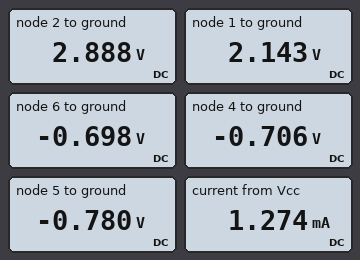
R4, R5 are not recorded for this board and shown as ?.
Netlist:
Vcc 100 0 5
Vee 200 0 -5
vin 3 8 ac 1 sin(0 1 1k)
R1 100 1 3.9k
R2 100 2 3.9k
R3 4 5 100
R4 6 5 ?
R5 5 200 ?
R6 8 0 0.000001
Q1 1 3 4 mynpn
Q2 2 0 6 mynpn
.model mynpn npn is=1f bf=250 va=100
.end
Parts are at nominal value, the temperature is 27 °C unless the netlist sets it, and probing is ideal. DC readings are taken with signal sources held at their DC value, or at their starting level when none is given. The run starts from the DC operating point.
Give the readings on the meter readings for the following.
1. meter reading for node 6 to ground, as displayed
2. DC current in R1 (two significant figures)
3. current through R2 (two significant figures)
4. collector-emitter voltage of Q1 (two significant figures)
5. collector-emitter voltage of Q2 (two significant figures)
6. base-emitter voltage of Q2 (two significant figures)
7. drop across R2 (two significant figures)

-0.698 V
730 µA
540 µA
2.8 V
3.6 V
700 mV
2.1 V
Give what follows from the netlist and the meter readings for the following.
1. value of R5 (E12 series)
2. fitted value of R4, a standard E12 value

3.3 kΩ
150 Ω
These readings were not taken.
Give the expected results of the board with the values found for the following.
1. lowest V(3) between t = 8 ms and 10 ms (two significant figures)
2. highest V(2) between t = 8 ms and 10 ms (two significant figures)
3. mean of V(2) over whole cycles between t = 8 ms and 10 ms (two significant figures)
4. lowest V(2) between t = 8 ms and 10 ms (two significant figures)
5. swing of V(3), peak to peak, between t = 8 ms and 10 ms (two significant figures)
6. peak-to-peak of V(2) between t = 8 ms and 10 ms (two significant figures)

-1.0 V
5.0 V
2.6 V
180 mV
2.0 V
4.8 V
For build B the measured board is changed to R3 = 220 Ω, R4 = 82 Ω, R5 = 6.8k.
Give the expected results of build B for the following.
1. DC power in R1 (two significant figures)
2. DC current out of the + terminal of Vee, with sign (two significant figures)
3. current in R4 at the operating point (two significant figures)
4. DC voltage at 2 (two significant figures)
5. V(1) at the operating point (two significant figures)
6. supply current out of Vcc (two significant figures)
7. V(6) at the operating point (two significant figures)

190 µW
-630 µA
410 µA
3.4 V
4.1 V
630 µA
-690 mV
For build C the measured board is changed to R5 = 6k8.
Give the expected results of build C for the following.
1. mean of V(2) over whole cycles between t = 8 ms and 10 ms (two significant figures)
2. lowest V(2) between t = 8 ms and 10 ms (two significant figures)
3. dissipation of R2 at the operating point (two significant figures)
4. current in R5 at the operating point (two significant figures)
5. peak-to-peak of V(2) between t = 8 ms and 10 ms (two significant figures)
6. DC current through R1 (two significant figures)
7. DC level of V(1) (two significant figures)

3.8 V
2.6 V
300 µW
630 µA
2.4 V
350 µA
3.6 V
